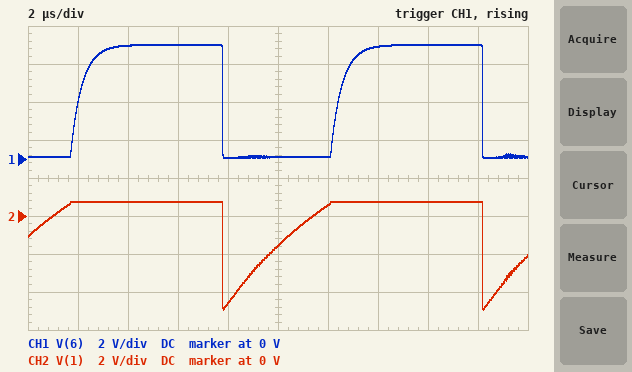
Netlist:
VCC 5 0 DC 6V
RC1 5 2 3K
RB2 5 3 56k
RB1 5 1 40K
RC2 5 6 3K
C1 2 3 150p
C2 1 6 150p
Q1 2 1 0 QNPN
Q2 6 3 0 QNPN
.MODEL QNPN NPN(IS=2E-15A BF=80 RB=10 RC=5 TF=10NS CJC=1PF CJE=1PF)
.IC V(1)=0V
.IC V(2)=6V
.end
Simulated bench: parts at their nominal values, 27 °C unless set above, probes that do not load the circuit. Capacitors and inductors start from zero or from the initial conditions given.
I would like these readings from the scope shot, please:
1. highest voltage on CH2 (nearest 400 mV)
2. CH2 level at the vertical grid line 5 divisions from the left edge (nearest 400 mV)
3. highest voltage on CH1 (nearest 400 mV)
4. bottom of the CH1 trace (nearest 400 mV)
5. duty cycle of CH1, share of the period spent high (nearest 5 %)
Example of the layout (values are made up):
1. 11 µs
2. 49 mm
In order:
1. 800 mV
2. -1.6 V
3. 6.0 V
4. 0 V
5. 55 %
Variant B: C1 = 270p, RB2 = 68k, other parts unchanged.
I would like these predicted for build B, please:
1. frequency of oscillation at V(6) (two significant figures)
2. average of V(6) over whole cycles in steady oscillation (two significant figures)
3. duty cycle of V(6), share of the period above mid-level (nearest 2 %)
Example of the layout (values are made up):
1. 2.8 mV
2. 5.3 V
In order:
1. 57 kHz
2. 4.4 V
3. 74 %
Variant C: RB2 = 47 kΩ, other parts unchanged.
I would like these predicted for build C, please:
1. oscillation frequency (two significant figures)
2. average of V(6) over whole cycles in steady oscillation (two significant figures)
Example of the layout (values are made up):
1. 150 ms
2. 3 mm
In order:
1. 110 kHz
2. 3.0 V
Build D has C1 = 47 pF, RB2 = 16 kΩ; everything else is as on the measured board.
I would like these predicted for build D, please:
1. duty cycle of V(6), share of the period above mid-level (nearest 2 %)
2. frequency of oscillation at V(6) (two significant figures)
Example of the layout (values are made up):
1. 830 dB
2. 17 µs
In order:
1. 10 %
2. 260 kHz
